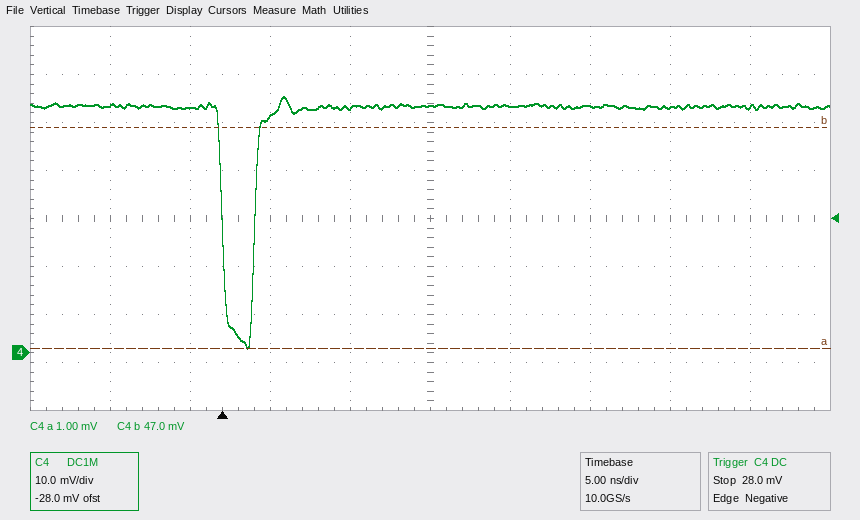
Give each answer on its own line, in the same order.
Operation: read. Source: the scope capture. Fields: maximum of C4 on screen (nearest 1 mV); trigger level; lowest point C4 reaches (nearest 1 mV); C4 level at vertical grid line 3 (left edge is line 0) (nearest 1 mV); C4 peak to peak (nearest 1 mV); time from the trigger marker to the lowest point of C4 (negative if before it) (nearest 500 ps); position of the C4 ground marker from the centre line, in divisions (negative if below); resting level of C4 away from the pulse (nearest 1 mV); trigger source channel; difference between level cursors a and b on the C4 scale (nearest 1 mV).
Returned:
53 mV
28.0 mV
1 mV
49 mV
52 mV
+1.5 ns
-2.8 div
51 mV
C4
46 mV
